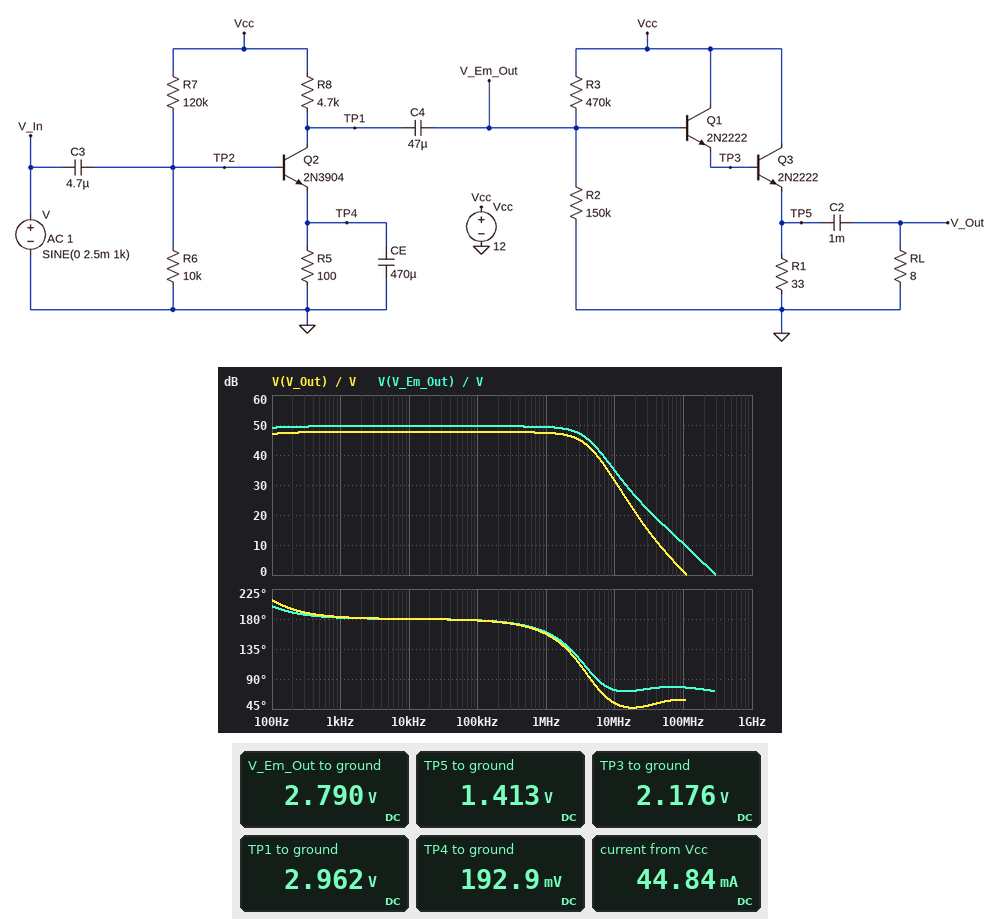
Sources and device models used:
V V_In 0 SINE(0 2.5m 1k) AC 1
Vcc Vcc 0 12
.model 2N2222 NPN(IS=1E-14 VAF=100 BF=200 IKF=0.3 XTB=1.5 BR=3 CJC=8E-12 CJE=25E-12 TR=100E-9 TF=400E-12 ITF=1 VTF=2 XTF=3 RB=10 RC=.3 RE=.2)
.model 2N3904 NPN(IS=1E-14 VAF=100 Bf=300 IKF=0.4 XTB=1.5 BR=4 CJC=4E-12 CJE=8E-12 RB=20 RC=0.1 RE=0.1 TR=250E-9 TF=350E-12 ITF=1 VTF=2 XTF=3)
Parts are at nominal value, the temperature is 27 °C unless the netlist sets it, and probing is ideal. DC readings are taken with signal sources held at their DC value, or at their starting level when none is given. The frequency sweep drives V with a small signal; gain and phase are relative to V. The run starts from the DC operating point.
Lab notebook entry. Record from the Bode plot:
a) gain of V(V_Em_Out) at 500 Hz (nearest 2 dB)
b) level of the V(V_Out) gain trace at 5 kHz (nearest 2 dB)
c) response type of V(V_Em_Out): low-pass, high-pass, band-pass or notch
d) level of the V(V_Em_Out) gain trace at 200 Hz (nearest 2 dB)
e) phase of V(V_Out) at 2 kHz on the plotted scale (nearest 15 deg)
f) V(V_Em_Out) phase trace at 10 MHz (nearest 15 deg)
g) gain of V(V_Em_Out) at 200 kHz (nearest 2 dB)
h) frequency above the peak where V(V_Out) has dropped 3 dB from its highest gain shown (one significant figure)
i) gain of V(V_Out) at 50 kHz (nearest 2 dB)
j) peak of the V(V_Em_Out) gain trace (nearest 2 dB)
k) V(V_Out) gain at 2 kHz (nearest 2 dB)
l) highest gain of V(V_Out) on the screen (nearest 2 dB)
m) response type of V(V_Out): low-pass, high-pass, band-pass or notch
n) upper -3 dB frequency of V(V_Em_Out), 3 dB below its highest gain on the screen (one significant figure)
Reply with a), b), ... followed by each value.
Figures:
a) 50 dB
b) 48 dB
c) low-pass
d) 50 dB
e) 180 deg
f) 75 deg
g) 50 dB
h) 3 MHz
i) 48 dB
j) 50 dB
k) 48 dB
l) 48 dB
m) low-pass
n) 3 MHz
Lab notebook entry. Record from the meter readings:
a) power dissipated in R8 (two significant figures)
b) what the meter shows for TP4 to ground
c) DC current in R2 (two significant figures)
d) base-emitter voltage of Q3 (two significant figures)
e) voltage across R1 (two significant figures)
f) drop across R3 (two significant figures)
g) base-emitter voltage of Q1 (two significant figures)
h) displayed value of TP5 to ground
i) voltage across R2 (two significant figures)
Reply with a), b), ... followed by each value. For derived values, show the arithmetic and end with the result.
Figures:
a) (12 V - 2.962 V)^2 / 4.7 kΩ = 17 mW
b) 192.9 mV
c) (2.79 V) / 150 kΩ = 19 µA
d) 2.176 V - 1.413 V = 760 mV
e) 1.413 V = 1.4 V
f) 12 V - 2.79 V = 9.2 V
g) 2.79 V - 2.176 V = 610 mV
h) 1.413 V
i) 2.79 V = 2.8 V
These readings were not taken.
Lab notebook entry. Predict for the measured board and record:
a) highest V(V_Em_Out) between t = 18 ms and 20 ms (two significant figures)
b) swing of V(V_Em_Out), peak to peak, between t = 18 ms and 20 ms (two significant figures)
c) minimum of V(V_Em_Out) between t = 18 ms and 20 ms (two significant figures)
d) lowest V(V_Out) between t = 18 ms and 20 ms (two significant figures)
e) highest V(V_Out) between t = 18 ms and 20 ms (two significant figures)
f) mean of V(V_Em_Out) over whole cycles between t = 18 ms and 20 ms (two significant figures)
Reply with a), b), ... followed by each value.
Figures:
a) 3.5 V
b) 1.5 V
c) 2.0 V
d) -300 mV
e) 530 mV
f) 2.8 V
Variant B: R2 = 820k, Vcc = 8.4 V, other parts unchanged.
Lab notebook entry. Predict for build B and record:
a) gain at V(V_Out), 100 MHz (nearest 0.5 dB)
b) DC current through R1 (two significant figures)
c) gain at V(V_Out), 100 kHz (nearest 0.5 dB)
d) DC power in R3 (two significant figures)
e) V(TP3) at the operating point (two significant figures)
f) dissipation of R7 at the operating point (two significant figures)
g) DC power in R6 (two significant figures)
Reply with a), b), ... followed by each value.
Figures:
a) -14.0 dB
b) 93 mA
c) 31.0 dB
d) 32 µW
e) 3.9 V
f) 500 µW
g) 41 µW
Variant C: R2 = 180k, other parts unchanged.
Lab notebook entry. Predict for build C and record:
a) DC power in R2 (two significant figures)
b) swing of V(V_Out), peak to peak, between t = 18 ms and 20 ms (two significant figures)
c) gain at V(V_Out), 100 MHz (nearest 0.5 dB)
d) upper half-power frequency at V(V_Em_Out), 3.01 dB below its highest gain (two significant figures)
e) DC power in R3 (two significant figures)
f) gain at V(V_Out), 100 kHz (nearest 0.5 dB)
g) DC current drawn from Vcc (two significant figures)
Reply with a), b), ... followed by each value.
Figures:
a) 55 µW
b) 920 mV
c) 1.5 dB
d) 3.5 MHz
e) 170 µW
f) 48.0 dB
g) 55 mA
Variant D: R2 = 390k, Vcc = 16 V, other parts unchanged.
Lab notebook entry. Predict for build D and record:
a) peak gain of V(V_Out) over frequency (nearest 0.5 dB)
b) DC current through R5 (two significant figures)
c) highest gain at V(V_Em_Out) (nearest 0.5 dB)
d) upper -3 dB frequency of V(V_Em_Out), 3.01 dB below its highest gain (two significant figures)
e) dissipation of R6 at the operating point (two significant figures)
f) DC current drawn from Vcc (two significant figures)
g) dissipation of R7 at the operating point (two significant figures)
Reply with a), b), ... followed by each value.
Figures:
a) 30.0 dB
b) 3.3 mA
c) 31.0 dB
d) 360 kHz
e) 100 µW
f) 150 mA
g) 1.9 mW
